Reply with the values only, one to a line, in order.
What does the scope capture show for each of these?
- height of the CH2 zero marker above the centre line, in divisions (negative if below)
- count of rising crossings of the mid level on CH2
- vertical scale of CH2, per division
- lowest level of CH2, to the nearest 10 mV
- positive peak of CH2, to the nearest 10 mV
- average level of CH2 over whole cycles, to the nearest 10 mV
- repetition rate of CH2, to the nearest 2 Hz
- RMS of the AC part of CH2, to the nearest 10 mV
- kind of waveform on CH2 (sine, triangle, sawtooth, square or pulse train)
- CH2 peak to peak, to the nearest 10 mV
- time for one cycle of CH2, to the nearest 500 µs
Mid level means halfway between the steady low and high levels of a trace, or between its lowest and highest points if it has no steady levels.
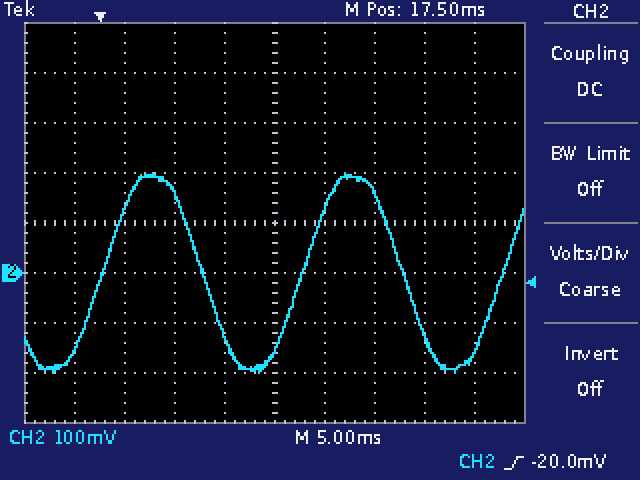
-1.0 div
3
100 mV
-200 mV
200 mV
0 mV
50 Hz
140 mV
sine
400 mV
20.0 ms
